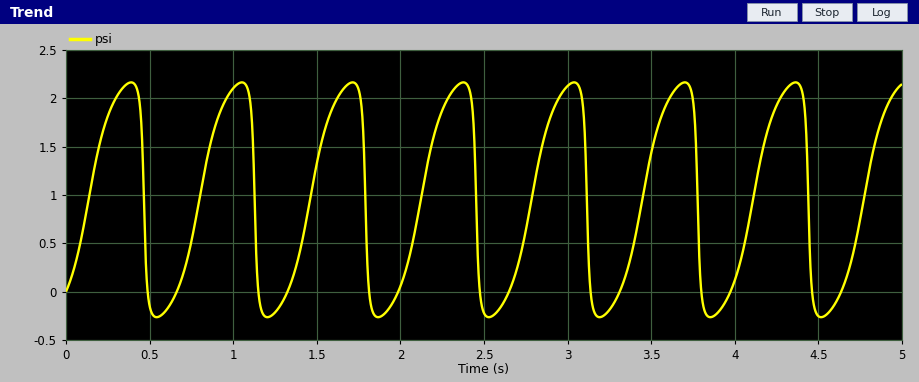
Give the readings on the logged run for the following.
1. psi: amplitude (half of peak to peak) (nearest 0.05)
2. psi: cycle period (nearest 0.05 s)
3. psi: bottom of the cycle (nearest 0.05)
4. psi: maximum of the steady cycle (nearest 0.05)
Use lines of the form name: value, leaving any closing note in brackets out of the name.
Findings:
psi: amplitude (half of peak to peak): 1.20
psi: cycle period: 0.65 s
psi: bottom of the cycle: -0.25
psi: maximum of the steady cycle: 2.15
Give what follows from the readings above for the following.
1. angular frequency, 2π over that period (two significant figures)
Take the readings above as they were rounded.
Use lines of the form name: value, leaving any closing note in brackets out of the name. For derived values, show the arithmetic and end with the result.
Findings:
angular frequency, 2π over that period: 2π / 0.65 = 9.7 rad/s
